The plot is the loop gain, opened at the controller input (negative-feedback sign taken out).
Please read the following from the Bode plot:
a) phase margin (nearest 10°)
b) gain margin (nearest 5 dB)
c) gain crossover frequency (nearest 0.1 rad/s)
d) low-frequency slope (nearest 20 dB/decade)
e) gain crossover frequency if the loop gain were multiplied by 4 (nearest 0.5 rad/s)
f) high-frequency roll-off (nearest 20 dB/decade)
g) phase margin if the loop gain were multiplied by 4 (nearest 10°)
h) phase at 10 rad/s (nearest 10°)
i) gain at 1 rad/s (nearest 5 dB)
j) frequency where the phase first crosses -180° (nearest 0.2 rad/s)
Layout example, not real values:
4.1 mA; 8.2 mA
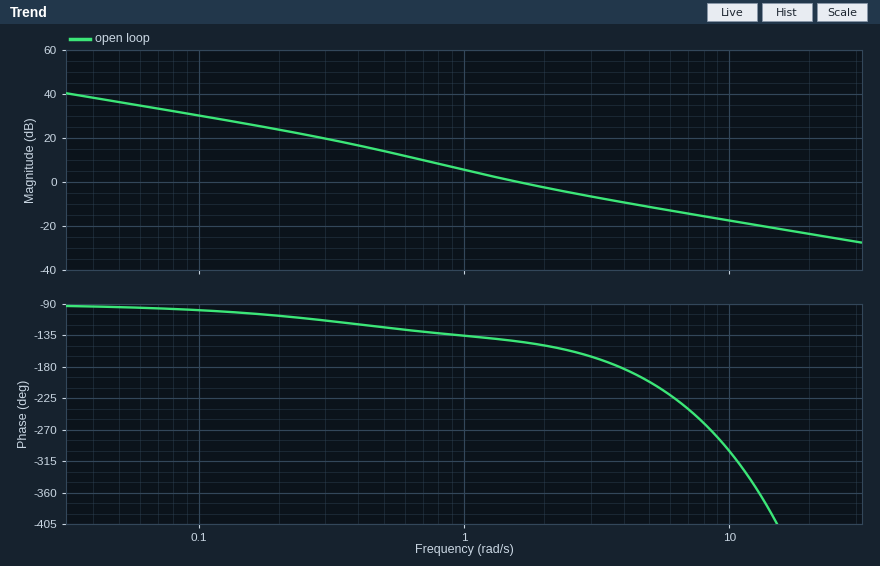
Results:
40°; 10 dB; 1.6 rad/s; -20 dB/decade; 5.5 rad/s; -20 dB/decade; -30°; -300°; 5 dB; 3.8 rad/s
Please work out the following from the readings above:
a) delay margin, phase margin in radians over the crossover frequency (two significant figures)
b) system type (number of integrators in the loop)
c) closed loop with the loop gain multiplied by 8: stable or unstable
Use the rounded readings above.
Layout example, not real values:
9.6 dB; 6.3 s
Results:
0.44 s; 1; unstable
